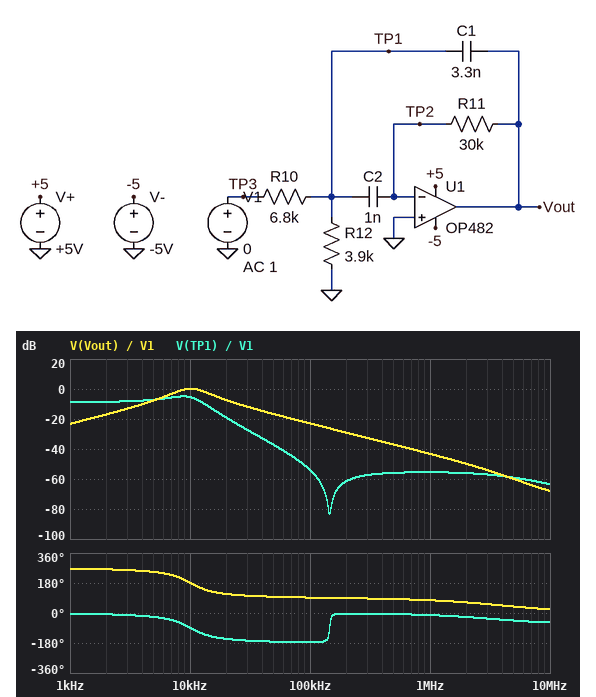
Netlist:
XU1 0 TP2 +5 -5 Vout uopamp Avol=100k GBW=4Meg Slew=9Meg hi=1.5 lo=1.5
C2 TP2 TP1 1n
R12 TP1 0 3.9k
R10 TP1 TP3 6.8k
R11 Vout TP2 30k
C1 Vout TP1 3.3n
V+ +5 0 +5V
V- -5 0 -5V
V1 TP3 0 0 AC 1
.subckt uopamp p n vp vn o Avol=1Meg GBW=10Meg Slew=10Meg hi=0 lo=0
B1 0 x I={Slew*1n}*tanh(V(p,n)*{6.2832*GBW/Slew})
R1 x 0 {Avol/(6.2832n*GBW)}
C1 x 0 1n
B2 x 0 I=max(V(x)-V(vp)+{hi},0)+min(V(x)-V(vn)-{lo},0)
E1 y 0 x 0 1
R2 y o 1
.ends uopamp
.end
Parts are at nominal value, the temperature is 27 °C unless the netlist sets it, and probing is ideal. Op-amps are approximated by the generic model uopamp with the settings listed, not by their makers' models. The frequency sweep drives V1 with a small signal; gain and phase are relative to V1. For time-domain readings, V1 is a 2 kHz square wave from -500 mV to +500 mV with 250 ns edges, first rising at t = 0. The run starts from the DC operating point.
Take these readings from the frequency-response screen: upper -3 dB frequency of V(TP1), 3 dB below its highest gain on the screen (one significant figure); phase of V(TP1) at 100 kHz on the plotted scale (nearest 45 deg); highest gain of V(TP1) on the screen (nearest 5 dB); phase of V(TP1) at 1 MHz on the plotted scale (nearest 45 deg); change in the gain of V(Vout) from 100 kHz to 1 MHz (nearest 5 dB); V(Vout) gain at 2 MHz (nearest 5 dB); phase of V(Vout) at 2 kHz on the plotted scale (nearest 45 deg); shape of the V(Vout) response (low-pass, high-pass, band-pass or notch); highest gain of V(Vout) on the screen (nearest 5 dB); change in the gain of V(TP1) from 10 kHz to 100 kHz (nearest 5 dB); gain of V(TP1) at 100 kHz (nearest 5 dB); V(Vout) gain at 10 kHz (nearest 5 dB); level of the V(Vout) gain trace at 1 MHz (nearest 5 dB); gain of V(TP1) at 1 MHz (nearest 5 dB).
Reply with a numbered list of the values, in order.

1. 10 kHz
2. -180 deg
3. -5 dB
4. 0 deg
5. -20 dB
6. -50 dB
7. 270 deg
8. band-pass
9. 0 dB
10. -50 dB
11. -55 dB
12. 0 dB
13. -45 dB
14. -55 dB
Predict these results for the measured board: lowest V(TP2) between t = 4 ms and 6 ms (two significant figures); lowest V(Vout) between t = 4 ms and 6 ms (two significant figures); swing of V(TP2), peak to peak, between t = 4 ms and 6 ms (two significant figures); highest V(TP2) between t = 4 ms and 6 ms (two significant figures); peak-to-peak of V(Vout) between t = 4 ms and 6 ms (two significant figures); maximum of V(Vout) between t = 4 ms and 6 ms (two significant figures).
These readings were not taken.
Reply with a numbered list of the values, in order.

1. -1.8 mV
2. -450 mV
3. 3.5 mV
4. 1.8 mV
5. 900 mV
6. 450 mV
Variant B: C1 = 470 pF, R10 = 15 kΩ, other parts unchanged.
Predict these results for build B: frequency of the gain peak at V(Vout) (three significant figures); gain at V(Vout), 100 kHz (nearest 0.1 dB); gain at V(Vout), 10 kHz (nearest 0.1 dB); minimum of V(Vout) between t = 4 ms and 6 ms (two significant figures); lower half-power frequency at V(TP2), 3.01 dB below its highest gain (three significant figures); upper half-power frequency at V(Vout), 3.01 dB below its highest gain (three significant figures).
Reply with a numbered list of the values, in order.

1. 23.8 kHz
2. -12.8 dB
3. -7.0 dB
4. -600 mV
5. 20.0 kHz
6. 33.2 kHz
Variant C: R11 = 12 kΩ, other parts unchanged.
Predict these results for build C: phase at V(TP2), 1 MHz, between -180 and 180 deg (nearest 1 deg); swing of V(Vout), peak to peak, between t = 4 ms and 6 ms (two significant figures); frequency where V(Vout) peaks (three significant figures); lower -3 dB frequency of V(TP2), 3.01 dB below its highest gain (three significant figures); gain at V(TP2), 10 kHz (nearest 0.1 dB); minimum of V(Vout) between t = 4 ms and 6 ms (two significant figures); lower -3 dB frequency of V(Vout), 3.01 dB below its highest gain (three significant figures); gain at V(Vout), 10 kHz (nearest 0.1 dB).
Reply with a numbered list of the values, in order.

1. -12 deg
2. 470 mV
3. 16.0 kHz
4. 13.9 kHz
5. -62.4 dB
6. -230 mV
7. 9.59 kHz
8. -10.4 dB
